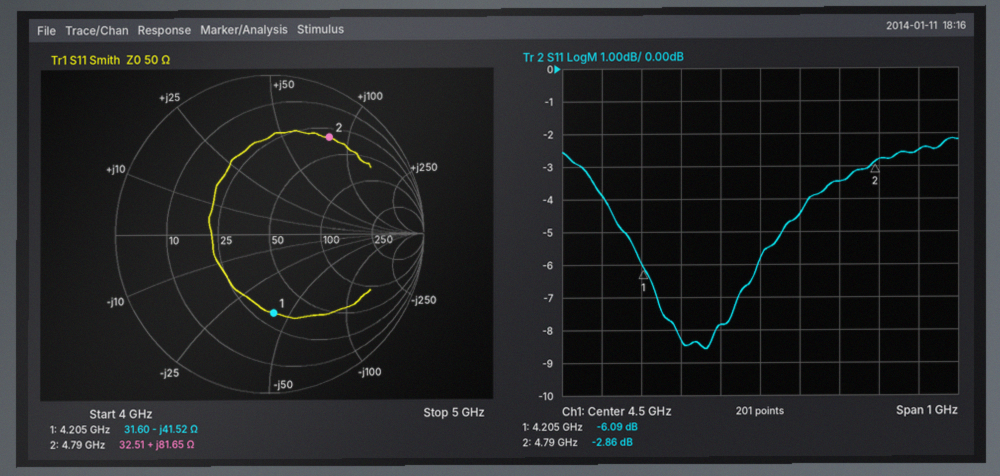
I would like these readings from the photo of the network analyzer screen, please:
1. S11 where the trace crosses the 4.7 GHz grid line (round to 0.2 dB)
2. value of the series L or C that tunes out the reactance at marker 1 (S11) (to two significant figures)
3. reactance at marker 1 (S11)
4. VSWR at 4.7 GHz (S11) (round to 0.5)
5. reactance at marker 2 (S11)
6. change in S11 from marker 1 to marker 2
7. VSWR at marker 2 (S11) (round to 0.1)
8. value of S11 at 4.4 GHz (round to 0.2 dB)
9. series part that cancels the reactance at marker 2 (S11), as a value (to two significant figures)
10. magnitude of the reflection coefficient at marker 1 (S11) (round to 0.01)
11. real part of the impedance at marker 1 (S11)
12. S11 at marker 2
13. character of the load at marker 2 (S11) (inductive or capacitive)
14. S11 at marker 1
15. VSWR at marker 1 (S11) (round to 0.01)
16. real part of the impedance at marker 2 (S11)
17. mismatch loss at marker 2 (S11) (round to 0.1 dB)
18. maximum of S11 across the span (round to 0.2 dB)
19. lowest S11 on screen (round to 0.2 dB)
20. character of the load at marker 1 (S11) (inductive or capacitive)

-3.4 dB
1.6 nH
-41.52 Ω
5.0
+81.65 Ω
3.23 dB
6.1
-7.8 dB
410 fF
0.50
31.60 Ω
-2.86 dB
inductive
-6.09 dB
2.97
32.51 Ω
3.2 dB
-2.2 dB
-8.6 dB
capacitive
